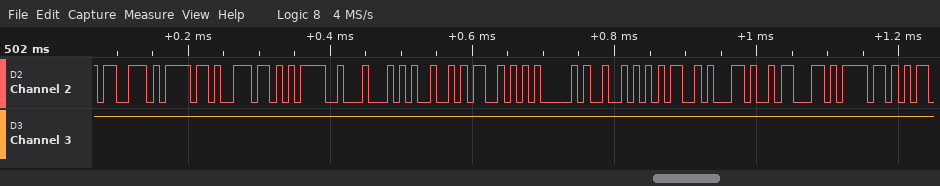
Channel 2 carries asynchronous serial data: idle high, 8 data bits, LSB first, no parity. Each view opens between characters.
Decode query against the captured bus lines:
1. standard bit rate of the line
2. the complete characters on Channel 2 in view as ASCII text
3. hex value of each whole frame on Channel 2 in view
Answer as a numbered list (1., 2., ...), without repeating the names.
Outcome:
1. 115200 baud
2. "son=DISARM,co"
3. 73, 6F, 6E, 3D, 44, 49, 53, 41, 52, 4D, 2C, 63, 6F
